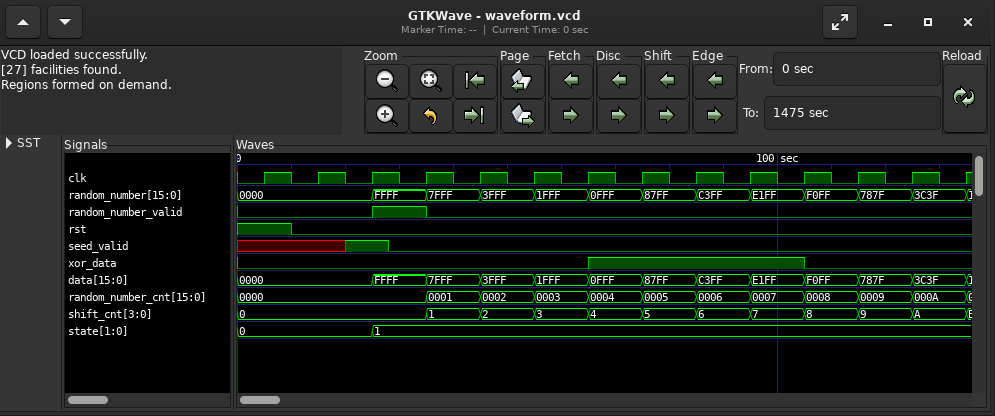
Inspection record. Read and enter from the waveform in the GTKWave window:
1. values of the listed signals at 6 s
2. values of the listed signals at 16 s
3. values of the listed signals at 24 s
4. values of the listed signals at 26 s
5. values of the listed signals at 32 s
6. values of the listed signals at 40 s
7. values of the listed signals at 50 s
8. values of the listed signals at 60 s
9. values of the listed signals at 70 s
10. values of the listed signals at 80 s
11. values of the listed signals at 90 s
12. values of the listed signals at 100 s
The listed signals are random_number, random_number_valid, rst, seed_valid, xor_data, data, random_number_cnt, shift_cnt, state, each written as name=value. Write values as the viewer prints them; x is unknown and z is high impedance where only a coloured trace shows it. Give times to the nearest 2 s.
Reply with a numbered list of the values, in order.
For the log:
1. random_number=0000, random_number_valid=0, rst=1, seed_valid=x, xor_data=0, data=0000, random_number_cnt=0000, shift_cnt=0, state=0
2. random_number=0000, random_number_valid=0, rst=0, seed_valid=x, xor_data=0, data=0000, random_number_cnt=0000, shift_cnt=0, state=0
3. random_number=0000, random_number_valid=0, rst=0, seed_valid=1, xor_data=0, data=0000, random_number_cnt=0000, shift_cnt=0, state=0
4. random_number=FFFF, random_number_valid=1, rst=0, seed_valid=1, xor_data=0, data=FFFF, random_number_cnt=0000, shift_cnt=0, state=1
5. random_number=FFFF, random_number_valid=1, rst=0, seed_valid=0, xor_data=0, data=FFFF, random_number_cnt=0000, shift_cnt=0, state=1
6. random_number=7FFF, random_number_valid=0, rst=0, seed_valid=0, xor_data=0, data=7FFF, random_number_cnt=0001, shift_cnt=1, state=1
7. random_number=3FFF, random_number_valid=0, rst=0, seed_valid=0, xor_data=0, data=3FFF, random_number_cnt=0002, shift_cnt=2, state=1
8. random_number=1FFF, random_number_valid=0, rst=0, seed_valid=0, xor_data=0, data=1FFF, random_number_cnt=0003, shift_cnt=3, state=1
9. random_number=0FFF, random_number_valid=0, rst=0, seed_valid=0, xor_data=1, data=0FFF, random_number_cnt=0004, shift_cnt=4, state=1
10. random_number=87FF, random_number_valid=0, rst=0, seed_valid=0, xor_data=1, data=87FF, random_number_cnt=0005, shift_cnt=5, state=1
11. random_number=C3FF, random_number_valid=0, rst=0, seed_valid=0, xor_data=1, data=C3FF, random_number_cnt=0006, shift_cnt=6, state=1
12. random_number=E1FF, random_number_valid=0, rst=0, seed_valid=0, xor_data=1, data=E1FF, random_number_cnt=0007, shift_cnt=7, state=1
